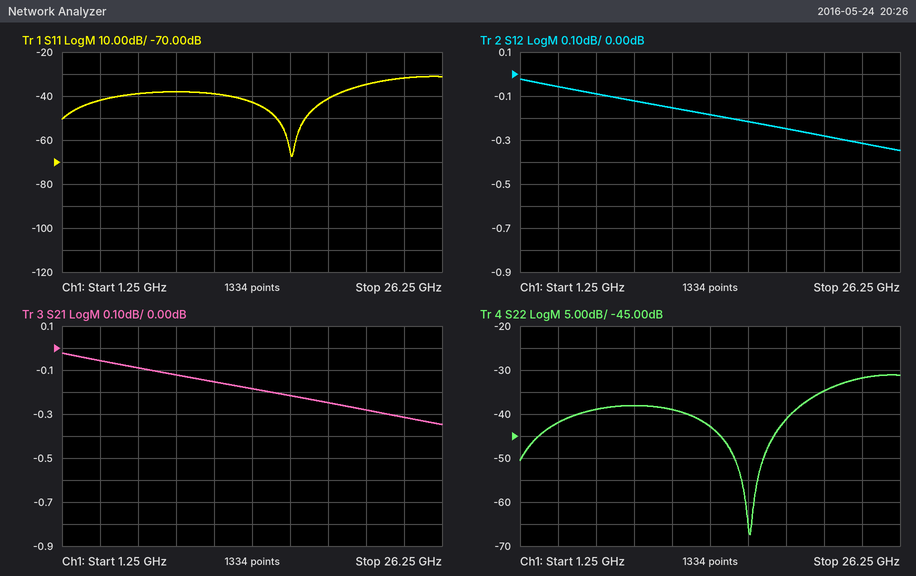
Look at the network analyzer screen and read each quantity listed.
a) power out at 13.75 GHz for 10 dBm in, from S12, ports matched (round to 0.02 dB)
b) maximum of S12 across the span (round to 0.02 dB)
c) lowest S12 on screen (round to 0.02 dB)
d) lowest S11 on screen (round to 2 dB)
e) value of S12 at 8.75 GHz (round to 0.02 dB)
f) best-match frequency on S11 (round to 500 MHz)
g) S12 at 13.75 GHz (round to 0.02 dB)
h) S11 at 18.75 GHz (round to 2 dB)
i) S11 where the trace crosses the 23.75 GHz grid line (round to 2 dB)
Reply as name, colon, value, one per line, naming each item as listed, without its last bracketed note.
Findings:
power out at 13.75 GHz for 10 dBm in, from S12, ports matched: 9.82 dBm
maximum of S12 across the span: -0.02 dB
lowest S12 on screen: -0.34 dB
lowest S11 on screen: -68 dB
value of S12 at 8.75 GHz: -0.12 dB
best-match frequency on S11: 16.5 GHz
S12 at 13.75 GHz: -0.18 dB
S11 at 18.75 GHz: -42 dB
S11 where the trace crosses the 23.75 GHz grid line: -32 dB
